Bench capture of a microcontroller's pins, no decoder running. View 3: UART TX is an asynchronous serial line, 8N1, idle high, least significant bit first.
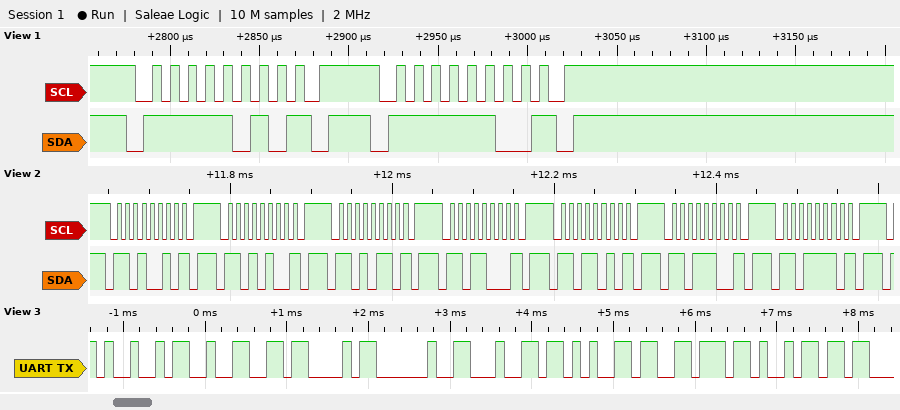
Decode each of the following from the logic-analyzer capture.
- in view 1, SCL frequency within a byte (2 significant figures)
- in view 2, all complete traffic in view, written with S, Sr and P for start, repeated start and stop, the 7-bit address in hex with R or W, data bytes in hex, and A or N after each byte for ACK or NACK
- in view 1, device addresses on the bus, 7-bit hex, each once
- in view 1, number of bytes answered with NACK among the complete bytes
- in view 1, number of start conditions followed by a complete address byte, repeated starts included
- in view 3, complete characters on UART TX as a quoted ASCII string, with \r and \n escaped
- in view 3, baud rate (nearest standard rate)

100 kHz
S 69W N P S 6AW N P S 6BW N P S 6CW N P S 6DW N P S 6EW N P S 6FW N P
0x7D 0x7E
2
2
"I2C devi"
9600 baud
